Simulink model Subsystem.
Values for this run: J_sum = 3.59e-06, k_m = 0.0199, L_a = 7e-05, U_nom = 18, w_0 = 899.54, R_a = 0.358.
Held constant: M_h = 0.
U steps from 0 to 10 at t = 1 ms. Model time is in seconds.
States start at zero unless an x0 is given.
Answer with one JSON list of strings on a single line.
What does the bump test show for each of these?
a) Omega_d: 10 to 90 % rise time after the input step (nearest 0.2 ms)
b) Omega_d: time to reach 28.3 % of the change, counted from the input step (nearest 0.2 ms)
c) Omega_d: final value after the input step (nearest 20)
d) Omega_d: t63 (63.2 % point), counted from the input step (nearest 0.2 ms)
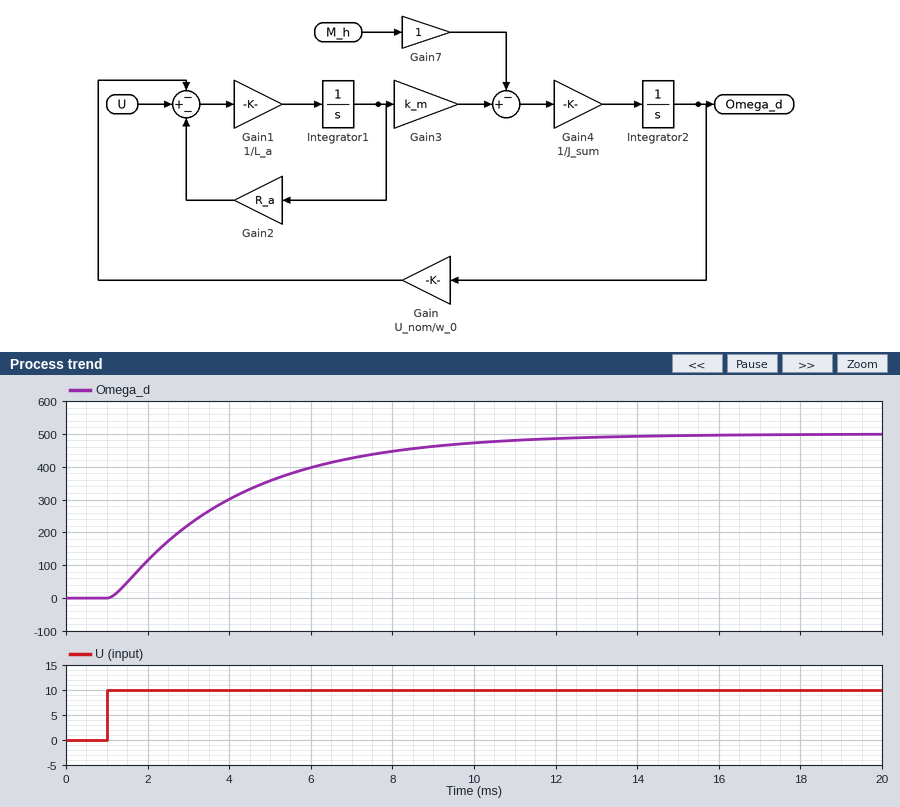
["6.6 ms", "1.2 ms", "500", "3.2 ms"]
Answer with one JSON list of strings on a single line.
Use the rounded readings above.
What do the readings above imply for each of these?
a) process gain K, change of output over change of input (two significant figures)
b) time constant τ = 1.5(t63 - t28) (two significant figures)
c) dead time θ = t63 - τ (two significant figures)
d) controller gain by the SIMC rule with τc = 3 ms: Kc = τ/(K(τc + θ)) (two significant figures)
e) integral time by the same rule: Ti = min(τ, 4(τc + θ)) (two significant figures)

["50", "3.0 ms", "0.20 ms", "0.019", "3.0 ms"]
